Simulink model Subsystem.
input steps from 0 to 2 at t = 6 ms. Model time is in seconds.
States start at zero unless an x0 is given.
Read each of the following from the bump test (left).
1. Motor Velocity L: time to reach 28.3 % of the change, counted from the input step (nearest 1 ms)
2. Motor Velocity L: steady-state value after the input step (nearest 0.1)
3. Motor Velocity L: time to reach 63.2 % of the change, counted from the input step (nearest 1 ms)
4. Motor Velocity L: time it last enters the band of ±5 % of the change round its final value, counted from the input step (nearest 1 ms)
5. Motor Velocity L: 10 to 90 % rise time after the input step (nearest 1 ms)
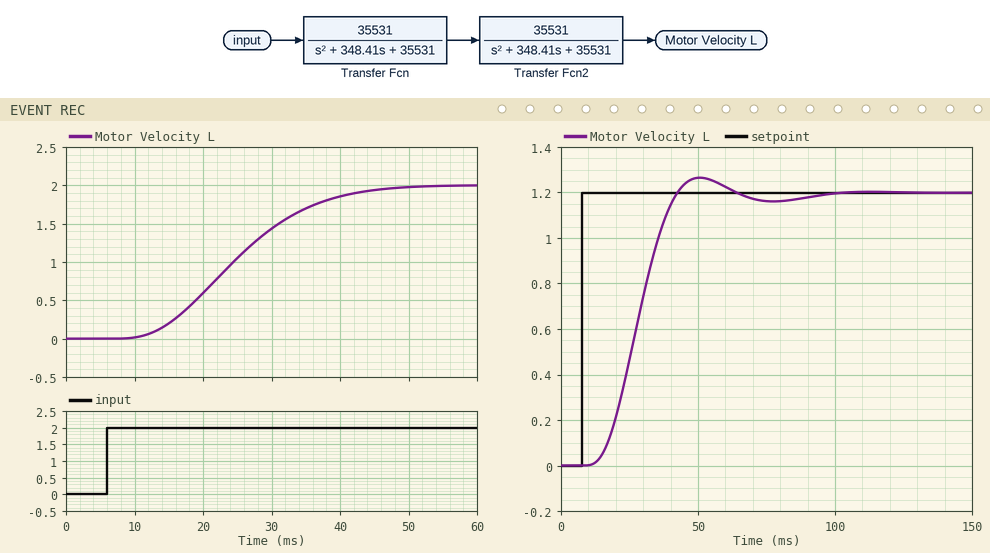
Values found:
14 ms
2.0
22 ms
36 ms
23 ms
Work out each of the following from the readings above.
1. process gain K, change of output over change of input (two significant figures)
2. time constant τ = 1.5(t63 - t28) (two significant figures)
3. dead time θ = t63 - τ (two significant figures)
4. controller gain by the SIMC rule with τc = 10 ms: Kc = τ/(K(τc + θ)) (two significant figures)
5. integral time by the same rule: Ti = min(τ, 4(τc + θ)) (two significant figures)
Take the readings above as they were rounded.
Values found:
1.0
12 ms
10 ms
0.60
12 ms
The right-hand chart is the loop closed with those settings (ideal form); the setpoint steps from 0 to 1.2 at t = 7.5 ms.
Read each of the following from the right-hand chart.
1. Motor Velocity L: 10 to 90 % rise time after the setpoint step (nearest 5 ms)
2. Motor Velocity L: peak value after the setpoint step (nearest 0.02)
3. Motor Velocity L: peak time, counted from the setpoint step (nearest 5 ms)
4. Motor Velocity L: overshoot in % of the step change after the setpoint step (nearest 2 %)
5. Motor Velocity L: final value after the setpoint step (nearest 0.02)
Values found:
20 ms
1.26
45 ms
6 %
1.20
